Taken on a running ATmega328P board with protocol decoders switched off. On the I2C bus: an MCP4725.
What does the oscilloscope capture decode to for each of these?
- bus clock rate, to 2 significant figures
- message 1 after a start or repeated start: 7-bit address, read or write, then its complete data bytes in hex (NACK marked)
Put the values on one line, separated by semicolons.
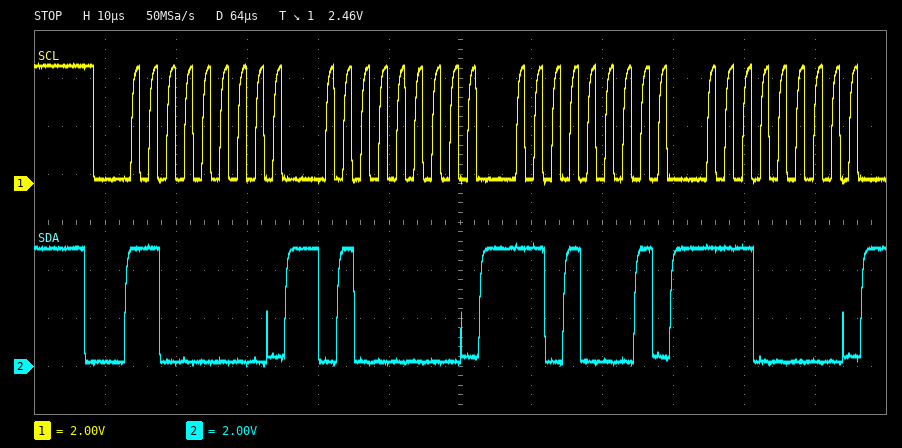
400 kHz; 0x60 write: 40 D1 E0
